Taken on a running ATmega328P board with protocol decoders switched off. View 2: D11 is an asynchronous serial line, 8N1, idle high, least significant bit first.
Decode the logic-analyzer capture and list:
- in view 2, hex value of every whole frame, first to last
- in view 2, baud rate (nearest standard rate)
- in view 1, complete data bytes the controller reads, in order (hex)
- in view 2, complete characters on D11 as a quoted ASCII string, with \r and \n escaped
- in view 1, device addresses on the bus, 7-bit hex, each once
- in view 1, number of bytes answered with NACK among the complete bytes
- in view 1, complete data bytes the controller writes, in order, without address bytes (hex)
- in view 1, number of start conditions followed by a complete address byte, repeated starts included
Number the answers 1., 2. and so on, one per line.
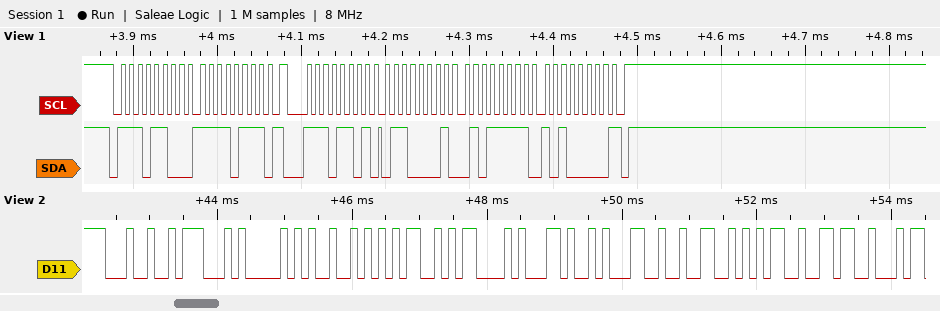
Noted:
1. 24 47 50 52 4D 43 2C 31 32 35 36
2. 9600 baud
3. 61 5F A0
4. "$GPRMC,1256"
5. 0x76
6. 1
7. F7
8. 2
